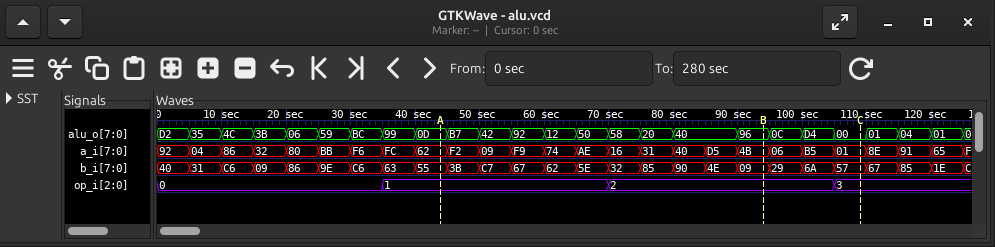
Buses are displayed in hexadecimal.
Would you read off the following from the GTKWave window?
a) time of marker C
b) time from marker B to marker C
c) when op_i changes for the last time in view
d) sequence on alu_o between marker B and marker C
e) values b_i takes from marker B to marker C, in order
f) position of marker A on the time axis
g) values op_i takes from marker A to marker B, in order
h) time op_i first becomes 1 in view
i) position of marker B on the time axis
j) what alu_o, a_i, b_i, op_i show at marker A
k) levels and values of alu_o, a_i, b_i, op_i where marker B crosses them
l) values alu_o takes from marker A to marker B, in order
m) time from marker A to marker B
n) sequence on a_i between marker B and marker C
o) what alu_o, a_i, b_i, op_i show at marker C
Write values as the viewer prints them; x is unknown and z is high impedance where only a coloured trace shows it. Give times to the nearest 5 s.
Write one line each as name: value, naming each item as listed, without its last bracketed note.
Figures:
time of marker C: 110 s
time from marker B to marker C: 15 s
when op_i changes for the last time in view: 105 s
sequence on alu_o between marker B and marker C: 96, 0C, D4, 00
values b_i takes from marker B to marker C, in order: 09, 29, 6A, 57
position of marker A on the time axis: 45 s
values op_i takes from marker A to marker B, in order: 1, 2
time op_i first becomes 1 in view: 35 s
position of marker B on the time axis: 95 s
what alu_o, a_i, b_i, op_i show at marker A: alu_o=0D, a_i=62, b_i=55, op_i=1
levels and values of alu_o, a_i, b_i, op_i where marker B crosses them: alu_o=96, a_i=4B, b_i=09, op_i=2
values alu_o takes from marker A to marker B, in order: 0D, B7, 42, 92, 12, 50, 58, 20, 40, 96
time from marker A to marker B: 50 s
sequence on a_i between marker B and marker C: 4B, 06, B5, 01
what alu_o, a_i, b_i, op_i show at marker C: alu_o=00, a_i=01, b_i=57, op_i=3
